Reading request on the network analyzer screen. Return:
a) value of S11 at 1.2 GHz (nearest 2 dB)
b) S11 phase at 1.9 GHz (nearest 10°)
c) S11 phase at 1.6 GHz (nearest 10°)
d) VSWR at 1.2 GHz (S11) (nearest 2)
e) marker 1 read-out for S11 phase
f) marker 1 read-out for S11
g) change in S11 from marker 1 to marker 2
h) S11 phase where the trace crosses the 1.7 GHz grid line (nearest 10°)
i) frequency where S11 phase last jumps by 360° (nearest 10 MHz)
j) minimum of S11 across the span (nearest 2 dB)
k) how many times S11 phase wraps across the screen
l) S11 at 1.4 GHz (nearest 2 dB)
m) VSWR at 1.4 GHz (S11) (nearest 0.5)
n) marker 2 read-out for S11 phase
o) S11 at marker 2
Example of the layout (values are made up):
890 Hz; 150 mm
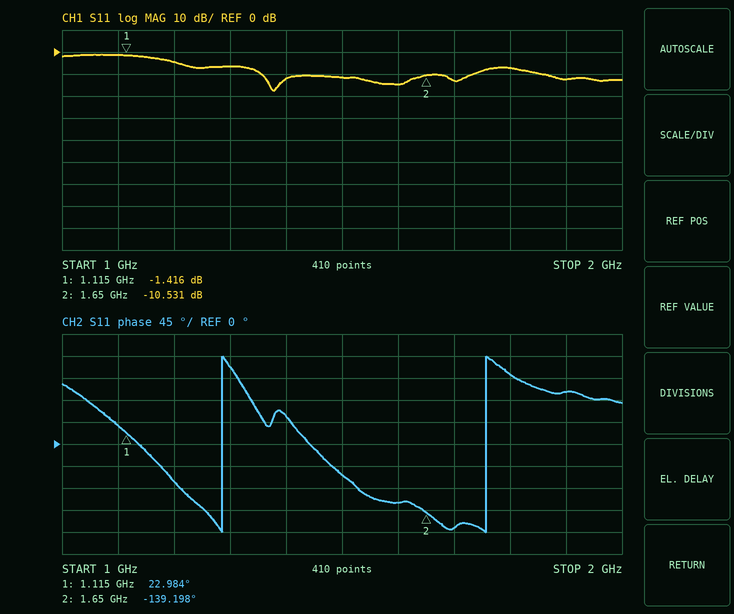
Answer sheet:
-4 dB; 110°; -120°; 4; 22.984°; -1.416 dB; -9.115 dB; -170°; 1.76 GHz; -18 dB; 2; -12 dB; 1.5; -139.198°; -10.531 dB
